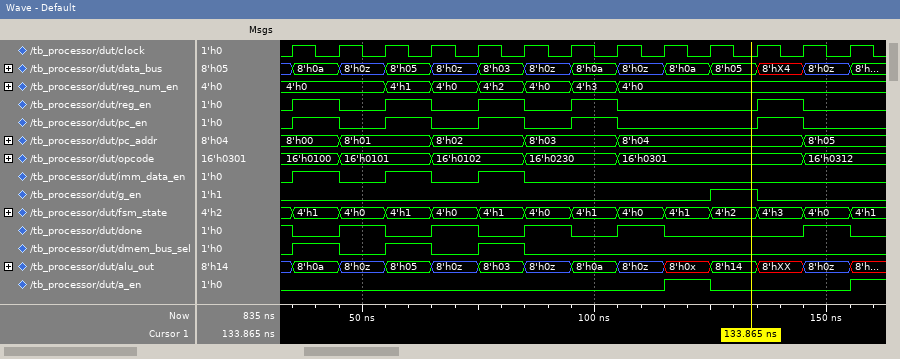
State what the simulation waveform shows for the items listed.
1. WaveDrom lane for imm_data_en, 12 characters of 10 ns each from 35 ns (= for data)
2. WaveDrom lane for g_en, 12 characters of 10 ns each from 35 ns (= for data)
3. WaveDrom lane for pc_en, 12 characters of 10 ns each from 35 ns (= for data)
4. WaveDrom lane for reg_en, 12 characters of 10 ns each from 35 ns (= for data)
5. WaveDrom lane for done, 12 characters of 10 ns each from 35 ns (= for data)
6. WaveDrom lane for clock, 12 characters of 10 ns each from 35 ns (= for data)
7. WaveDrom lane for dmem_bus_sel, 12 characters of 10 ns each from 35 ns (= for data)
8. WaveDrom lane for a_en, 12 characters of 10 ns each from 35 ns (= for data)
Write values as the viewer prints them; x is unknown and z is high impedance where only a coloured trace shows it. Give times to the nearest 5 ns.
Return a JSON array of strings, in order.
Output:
["{name: 'imm_data_en', wave: '101010......'}", "{name: 'g_en', wave: '0........10.'}", "{name: 'pc_en', wave: '10101010..10'}", "{name: 'reg_en', wave: '10101010..10'}", "{name: 'done', wave: '010101010..1'}", "{name: 'clock', wave: 'p...........'}", "{name: 'dmem_bus_sel', wave: '101010......'}", "{name: 'a_en', wave: '0.......10..'}"]
